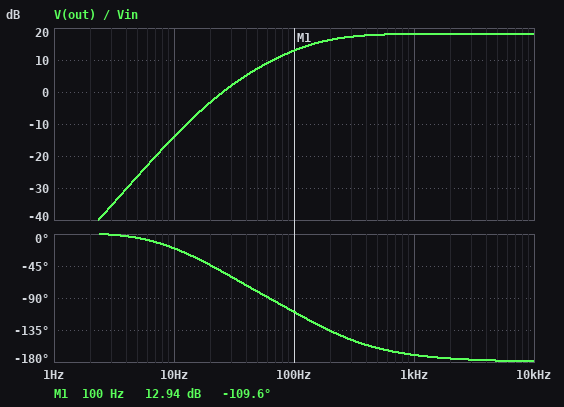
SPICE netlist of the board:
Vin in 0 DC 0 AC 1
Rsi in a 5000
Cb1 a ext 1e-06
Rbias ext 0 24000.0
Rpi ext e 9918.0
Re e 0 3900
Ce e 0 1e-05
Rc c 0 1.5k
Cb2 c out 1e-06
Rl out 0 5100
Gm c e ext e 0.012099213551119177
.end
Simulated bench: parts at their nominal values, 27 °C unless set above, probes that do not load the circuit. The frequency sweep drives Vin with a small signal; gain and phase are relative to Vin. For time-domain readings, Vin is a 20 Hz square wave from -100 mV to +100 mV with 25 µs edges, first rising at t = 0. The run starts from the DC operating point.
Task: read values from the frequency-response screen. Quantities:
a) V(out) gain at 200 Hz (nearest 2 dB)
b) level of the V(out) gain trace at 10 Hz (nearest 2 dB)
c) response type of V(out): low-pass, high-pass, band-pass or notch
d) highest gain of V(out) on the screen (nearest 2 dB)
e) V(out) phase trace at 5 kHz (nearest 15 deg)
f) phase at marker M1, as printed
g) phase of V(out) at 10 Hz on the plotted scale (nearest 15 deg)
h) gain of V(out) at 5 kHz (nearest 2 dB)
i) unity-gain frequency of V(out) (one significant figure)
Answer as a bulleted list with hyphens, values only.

- 16 dB
- -14 dB
- high-pass
- 18 dB
- -180 deg
- -109.6 deg
- -15 deg
- 18 dB
- 30 Hz
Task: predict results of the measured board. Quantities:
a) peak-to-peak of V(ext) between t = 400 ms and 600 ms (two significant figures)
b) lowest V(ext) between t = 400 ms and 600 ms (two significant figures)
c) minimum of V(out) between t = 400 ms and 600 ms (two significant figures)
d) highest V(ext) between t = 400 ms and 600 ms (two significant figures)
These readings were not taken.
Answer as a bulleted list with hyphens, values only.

- 190 mV
- -97 mV
- -1.6 V
- 97 mV
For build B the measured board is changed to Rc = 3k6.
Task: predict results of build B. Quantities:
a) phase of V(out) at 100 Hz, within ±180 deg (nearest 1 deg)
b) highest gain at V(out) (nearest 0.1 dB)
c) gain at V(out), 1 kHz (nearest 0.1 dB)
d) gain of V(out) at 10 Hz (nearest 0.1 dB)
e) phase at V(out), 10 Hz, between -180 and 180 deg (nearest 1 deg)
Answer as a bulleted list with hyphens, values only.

- -113 deg
- 23.5 dB
- 23.4 dB
- -6.8 dB
- -26 deg
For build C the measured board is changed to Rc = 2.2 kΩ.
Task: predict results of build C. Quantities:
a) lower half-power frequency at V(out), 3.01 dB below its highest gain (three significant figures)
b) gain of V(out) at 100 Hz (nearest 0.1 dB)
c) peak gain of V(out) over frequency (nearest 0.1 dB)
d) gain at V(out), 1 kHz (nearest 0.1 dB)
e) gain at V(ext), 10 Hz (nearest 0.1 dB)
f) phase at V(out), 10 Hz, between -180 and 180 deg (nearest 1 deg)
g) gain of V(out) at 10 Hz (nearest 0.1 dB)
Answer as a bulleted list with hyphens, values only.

- 152 Hz
- 15.4 dB
- 20.7 dB
- 20.6 dB
- -3.3 dB
- -22 deg
- -10.8 dB
